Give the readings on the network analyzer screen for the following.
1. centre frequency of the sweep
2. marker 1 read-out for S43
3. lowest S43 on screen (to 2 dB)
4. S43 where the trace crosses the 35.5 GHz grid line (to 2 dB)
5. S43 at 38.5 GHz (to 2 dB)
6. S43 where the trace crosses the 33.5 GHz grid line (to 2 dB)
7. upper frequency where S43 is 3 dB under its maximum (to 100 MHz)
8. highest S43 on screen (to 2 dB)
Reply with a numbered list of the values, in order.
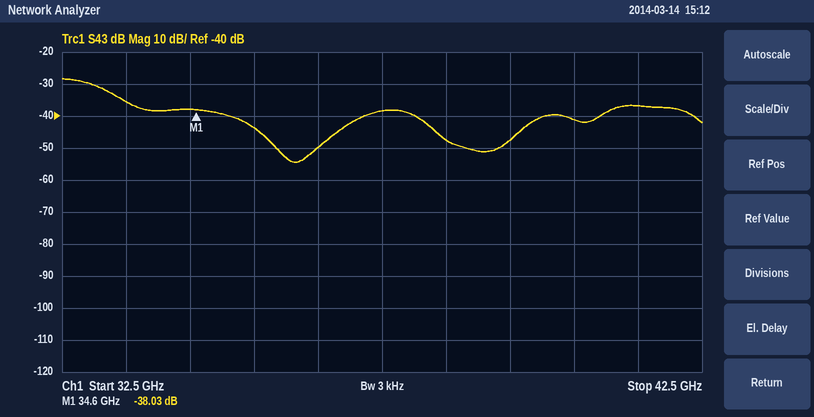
1. 37.5 GHz
2. -38.03 dB
3. -54 dB
4. -44 dB
5. -48 dB
6. -36 dB
7. 33.1 GHz
8. -28 dB
